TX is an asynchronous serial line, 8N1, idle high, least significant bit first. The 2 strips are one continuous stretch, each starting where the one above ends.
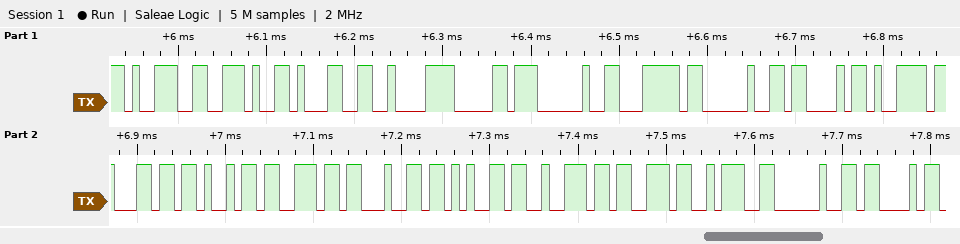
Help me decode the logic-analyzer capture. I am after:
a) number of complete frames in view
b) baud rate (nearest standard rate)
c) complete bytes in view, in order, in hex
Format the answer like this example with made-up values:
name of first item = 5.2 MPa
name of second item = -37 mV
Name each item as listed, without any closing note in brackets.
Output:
number of complete frames in view = 20
baud rate = 115200 baud
complete bytes in view, in order, in hex = 39 2E 31 C2 B0 20 7C 20 43 79 6C 69 6E 64 65 72 73 3A 20 43
